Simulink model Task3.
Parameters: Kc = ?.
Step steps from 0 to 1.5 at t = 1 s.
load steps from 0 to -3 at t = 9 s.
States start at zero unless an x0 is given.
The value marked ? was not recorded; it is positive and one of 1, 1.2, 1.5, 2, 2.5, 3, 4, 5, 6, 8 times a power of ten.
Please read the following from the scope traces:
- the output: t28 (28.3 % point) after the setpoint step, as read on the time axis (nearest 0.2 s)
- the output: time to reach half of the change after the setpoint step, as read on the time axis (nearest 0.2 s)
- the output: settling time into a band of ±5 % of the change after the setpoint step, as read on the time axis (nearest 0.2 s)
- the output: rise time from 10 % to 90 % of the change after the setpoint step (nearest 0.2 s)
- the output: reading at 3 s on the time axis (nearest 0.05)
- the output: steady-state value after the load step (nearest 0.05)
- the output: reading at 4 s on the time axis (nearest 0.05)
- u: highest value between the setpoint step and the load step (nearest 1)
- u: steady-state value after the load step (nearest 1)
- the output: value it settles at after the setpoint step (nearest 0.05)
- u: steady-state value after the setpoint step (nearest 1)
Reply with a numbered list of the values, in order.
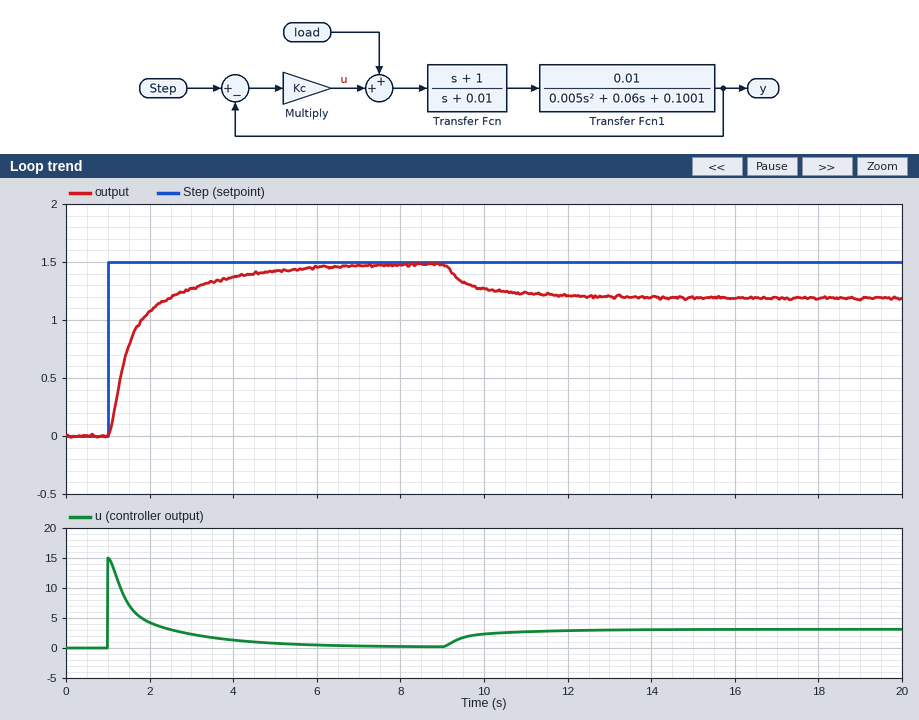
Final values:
1. 1.2 s
2. 1.4 s
3. 4.8 s
4. 2.4 s
5. 1.25
6. 1.20
7. 1.35
8. 15
9. 3
10. 1.50
11. 0
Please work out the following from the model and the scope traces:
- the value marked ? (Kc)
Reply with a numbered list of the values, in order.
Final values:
1. 10
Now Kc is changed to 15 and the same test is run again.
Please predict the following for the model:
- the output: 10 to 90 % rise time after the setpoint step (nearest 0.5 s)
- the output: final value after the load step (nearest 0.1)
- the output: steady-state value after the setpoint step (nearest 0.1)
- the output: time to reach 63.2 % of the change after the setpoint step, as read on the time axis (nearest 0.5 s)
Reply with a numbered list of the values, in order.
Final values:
1. 1.5 s
2. 1.3
3. 1.5
4. 1.5 s
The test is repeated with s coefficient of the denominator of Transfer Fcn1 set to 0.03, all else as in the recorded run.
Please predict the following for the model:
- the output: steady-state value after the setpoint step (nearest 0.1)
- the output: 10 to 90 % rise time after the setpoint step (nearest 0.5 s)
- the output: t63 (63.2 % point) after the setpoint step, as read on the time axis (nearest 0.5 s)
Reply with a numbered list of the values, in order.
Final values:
1. 1.5
2. 3.0 s
3. 1.5 s
